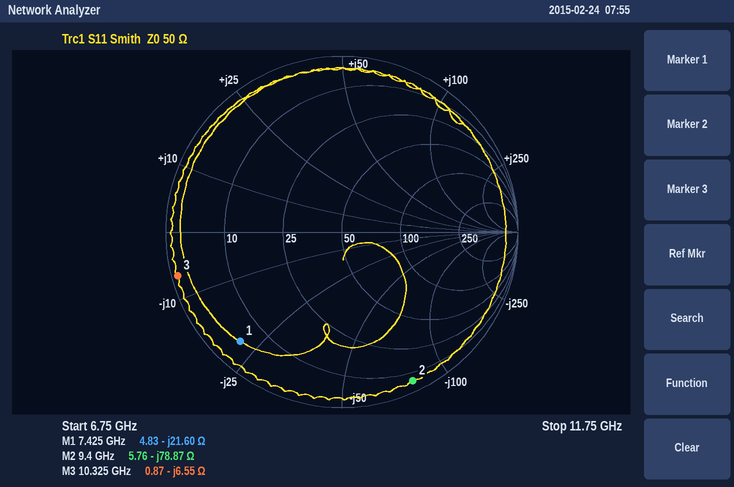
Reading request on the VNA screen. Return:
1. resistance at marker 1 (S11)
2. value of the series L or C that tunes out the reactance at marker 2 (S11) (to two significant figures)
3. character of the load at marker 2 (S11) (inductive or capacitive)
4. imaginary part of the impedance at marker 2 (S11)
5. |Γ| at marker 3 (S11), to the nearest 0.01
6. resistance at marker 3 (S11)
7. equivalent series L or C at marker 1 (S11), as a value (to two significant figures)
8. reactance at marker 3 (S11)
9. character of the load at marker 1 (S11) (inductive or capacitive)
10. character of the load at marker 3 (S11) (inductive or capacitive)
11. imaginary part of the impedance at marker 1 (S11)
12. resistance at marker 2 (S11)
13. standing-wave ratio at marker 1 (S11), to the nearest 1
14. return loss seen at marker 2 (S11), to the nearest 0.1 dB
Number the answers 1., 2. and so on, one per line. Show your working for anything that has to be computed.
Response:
1. 4.83 Ω
2. L = 78.87 Ω/(2π × 9.4 GHz) ≈ 1.3 nH
3. capacitive
4. -78.87 Ω
5. 0.97
6. 0.87 Ω
7. C = 1/(2π × 7.425 GHz × 21.6 Ω) ≈ 992 fF, so 990 fF to two significant figures
8. -6.55 Ω
9. capacitive
10. capacitive
11. -21.60 Ω
12. 5.76 Ω
13. 12
14. 0.6 dB
